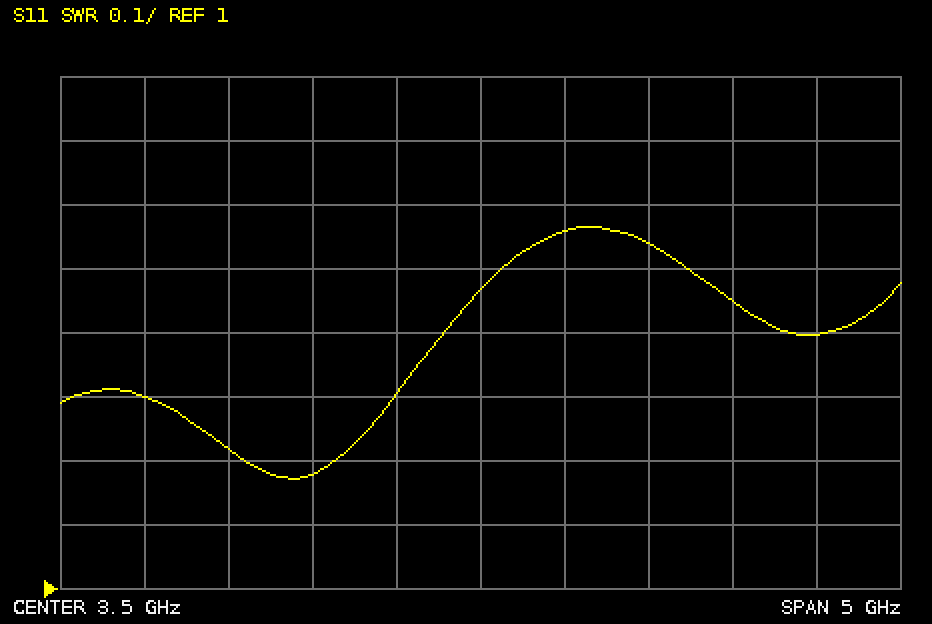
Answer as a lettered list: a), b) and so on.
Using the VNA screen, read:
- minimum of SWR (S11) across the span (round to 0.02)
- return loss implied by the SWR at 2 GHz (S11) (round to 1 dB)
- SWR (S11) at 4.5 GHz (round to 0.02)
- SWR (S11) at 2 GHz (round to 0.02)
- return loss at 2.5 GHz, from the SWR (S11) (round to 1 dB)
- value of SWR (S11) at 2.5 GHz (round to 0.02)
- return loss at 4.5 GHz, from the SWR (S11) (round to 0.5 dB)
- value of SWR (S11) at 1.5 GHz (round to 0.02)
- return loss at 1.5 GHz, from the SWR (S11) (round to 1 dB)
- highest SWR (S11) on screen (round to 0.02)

a) 1.18
b) 20 dB
c) 1.54
d) 1.22
e) 22 dB
f) 1.18
g) 13.5 dB
h) 1.30
i) 18 dB
j) 1.56
